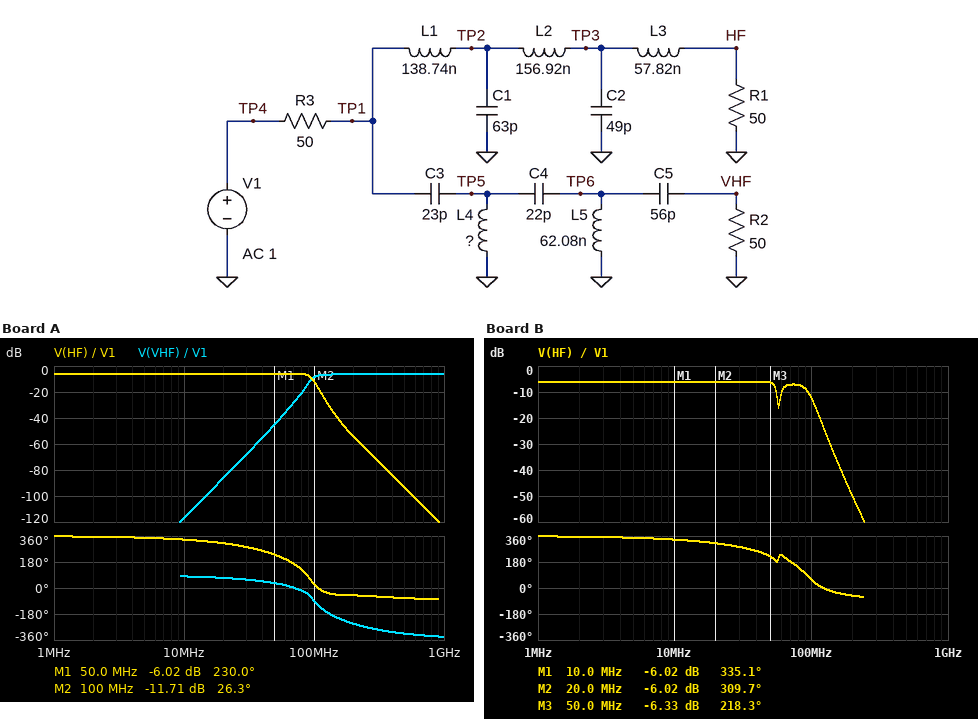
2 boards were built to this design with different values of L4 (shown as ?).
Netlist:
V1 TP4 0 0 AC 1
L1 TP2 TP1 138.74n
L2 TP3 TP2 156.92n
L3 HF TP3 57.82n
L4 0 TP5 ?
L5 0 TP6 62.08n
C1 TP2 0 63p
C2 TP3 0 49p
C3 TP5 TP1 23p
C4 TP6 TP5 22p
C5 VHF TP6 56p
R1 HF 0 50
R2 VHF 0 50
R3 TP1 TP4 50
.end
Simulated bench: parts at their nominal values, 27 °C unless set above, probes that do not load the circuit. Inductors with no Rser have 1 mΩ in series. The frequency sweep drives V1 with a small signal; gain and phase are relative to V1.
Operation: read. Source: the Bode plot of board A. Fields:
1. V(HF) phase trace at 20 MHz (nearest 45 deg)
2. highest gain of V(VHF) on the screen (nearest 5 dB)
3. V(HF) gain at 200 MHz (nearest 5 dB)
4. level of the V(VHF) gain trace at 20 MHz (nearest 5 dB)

315 deg
-5 dB
-55 dB
-85 dB
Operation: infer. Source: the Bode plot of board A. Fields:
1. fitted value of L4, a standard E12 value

33 nH
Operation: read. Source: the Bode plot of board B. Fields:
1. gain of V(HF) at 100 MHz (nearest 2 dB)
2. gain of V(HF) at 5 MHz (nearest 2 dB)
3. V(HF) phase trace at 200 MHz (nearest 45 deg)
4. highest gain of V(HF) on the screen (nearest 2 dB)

-12 dB
-6 dB
-45 deg
-6 dB
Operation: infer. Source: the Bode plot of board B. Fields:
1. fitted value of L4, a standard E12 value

150 nH
